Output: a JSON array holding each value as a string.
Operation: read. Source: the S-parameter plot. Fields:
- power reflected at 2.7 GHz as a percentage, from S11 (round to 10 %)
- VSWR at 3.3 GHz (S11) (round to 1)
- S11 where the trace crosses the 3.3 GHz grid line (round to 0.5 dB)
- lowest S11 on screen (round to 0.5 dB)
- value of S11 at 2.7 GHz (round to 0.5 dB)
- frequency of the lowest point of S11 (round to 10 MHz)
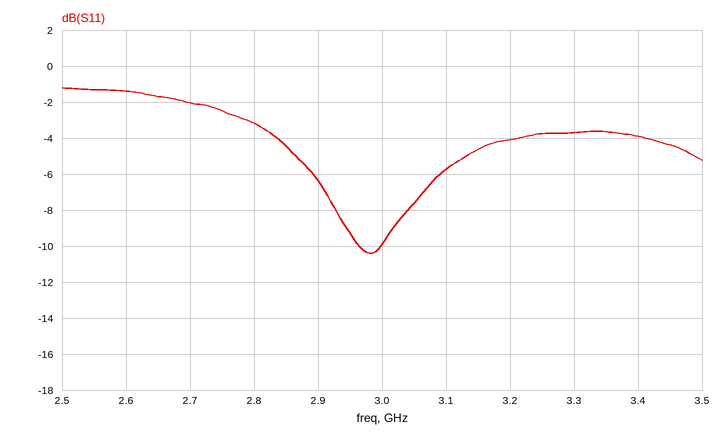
["60 %", "5", "-3.5 dB", "-10.5 dB", "-2.0 dB", "2.98 GHz"]
